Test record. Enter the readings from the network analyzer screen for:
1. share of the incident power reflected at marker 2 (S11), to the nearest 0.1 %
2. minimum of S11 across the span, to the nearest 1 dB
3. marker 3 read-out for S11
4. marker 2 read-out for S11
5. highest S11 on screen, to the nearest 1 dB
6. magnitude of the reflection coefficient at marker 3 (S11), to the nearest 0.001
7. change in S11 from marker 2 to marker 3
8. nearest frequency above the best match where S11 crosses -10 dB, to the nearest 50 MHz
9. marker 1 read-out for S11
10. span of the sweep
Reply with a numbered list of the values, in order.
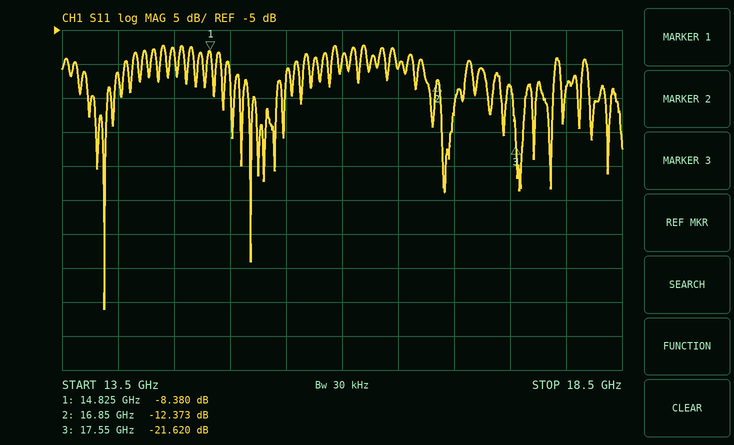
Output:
1. 5.8 %
2. -46 dB
3. -21.620 dB
4. -12.373 dB
5. -7 dB
6. 0.083
7. -9.247 dB
8. 14.05 GHz
9. -8.380 dB
10. 5 GHz
